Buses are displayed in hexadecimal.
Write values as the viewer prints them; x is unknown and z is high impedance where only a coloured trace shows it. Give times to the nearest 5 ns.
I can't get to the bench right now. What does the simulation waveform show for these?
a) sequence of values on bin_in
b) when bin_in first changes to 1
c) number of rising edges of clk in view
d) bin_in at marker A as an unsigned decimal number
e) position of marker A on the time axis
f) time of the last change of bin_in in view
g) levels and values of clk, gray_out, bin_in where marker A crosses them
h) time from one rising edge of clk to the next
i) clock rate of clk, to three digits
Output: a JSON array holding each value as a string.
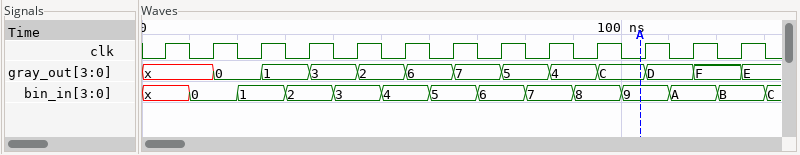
["x, 0, 1, 2, 3, 4, 5, 6, 7, 8, 9, A, B, C", "20 ns", "13", "9", "105 ns", "130 ns", "clk=0, gray_out=C, bin_in=9", "10 ns", "100 MHz"]
